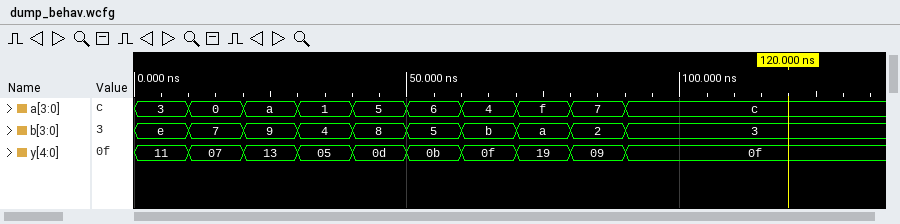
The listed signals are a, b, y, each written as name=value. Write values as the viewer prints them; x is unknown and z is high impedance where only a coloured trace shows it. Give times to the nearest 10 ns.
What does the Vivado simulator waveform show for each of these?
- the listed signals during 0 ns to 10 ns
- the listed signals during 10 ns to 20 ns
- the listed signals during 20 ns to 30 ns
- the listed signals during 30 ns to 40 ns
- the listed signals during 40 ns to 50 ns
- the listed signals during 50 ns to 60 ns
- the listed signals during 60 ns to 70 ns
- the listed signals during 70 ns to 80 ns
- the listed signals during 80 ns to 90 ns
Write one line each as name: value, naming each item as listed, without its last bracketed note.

the listed signals during 0 ns to 10 ns: a=3, b=e, y=11
the listed signals during 10 ns to 20 ns: a=0, b=7, y=07
the listed signals during 20 ns to 30 ns: a=a, b=9, y=13
the listed signals during 30 ns to 40 ns: a=1, b=4, y=05
the listed signals during 40 ns to 50 ns: a=5, b=8, y=0d
the listed signals during 50 ns to 60 ns: a=6, b=5, y=0b
the listed signals during 60 ns to 70 ns: a=4, b=b, y=0f
the listed signals during 70 ns to 80 ns: a=f, b=a, y=19
the listed signals during 80 ns to 90 ns: a=7, b=2, y=09
